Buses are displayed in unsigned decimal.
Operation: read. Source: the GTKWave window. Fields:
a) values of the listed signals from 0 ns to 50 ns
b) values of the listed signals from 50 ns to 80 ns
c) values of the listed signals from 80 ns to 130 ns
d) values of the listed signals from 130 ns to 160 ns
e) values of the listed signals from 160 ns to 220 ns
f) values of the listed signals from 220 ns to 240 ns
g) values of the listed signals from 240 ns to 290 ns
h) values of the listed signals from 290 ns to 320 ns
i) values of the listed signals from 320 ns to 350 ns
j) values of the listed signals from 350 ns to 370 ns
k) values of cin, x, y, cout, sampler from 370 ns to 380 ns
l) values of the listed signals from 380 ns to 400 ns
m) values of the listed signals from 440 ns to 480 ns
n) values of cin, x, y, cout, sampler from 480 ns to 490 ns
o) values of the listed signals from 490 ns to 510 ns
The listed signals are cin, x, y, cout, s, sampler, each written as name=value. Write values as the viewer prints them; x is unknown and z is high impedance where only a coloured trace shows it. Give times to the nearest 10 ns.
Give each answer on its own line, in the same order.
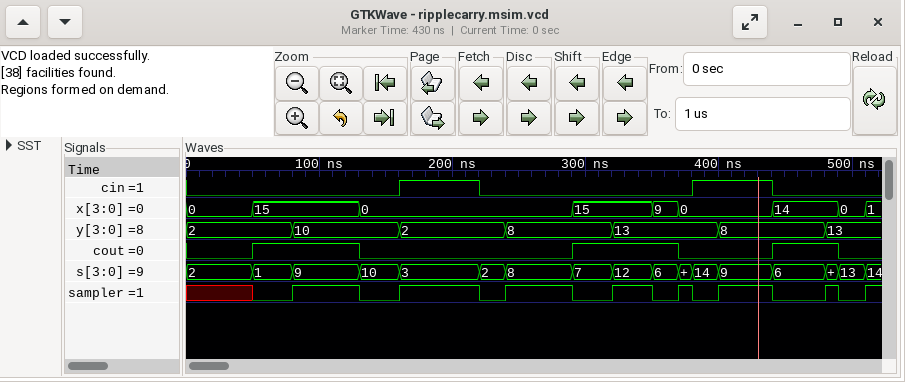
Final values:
cin=0, x=0, y=2, cout=0, s=2, sampler=x
cin=0, x=15, y=2, cout=1, s=1, sampler=0
cin=0, x=15, y=10, cout=1, s=9, sampler=1
cin=0, x=0, y=10, cout=0, s=10, sampler=0
cin=1, x=0, y=2, cout=0, s=3, sampler=1
cin=0, x=0, y=2, cout=0, s=2, sampler=0
cin=0, x=0, y=8, cout=0, s=8, sampler=1
cin=0, x=15, y=8, cout=1, s=7, sampler=0
cin=0, x=15, y=13, cout=1, s=12, sampler=1
cin=0, x=9, y=13, cout=1, s=6, sampler=0
cin=0, x=0, y=13, cout=0, sampler=1
cin=1, x=0, y=13, cout=0, s=14, sampler=0
cin=0, x=14, y=8, cout=1, s=6, sampler=0
cin=0, x=14, y=13, cout=1, sampler=1
cin=0, x=0, y=13, cout=0, s=13, sampler=0
